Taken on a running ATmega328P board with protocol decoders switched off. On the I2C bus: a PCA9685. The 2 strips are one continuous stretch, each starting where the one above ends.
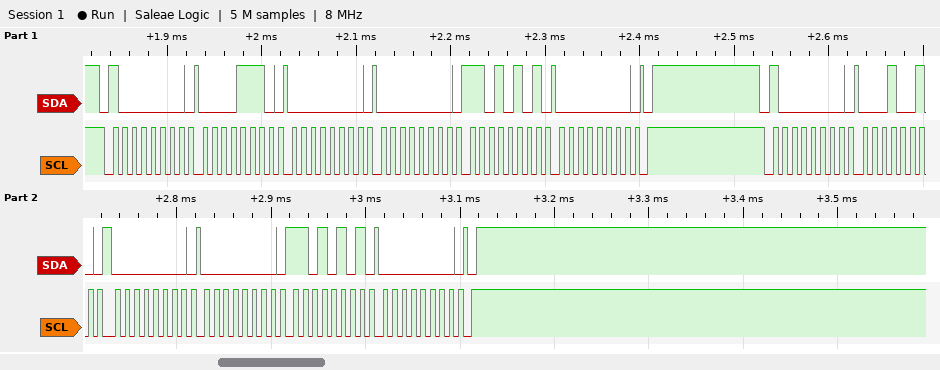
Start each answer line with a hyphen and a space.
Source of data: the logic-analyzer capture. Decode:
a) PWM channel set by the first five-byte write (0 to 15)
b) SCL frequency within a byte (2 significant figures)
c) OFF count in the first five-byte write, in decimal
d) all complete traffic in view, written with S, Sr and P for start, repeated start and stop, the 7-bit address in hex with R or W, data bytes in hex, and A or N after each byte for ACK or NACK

- 2
- 100 kHz
- 213
- S 40W A 0E A 00 A 00 A D5 A 00 A P S 40W A 12 A 00 A 00 A D5 A 00 A P
